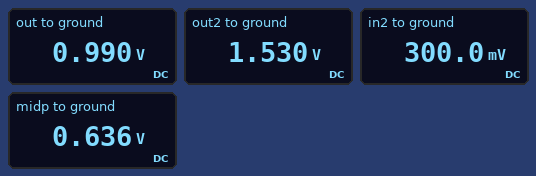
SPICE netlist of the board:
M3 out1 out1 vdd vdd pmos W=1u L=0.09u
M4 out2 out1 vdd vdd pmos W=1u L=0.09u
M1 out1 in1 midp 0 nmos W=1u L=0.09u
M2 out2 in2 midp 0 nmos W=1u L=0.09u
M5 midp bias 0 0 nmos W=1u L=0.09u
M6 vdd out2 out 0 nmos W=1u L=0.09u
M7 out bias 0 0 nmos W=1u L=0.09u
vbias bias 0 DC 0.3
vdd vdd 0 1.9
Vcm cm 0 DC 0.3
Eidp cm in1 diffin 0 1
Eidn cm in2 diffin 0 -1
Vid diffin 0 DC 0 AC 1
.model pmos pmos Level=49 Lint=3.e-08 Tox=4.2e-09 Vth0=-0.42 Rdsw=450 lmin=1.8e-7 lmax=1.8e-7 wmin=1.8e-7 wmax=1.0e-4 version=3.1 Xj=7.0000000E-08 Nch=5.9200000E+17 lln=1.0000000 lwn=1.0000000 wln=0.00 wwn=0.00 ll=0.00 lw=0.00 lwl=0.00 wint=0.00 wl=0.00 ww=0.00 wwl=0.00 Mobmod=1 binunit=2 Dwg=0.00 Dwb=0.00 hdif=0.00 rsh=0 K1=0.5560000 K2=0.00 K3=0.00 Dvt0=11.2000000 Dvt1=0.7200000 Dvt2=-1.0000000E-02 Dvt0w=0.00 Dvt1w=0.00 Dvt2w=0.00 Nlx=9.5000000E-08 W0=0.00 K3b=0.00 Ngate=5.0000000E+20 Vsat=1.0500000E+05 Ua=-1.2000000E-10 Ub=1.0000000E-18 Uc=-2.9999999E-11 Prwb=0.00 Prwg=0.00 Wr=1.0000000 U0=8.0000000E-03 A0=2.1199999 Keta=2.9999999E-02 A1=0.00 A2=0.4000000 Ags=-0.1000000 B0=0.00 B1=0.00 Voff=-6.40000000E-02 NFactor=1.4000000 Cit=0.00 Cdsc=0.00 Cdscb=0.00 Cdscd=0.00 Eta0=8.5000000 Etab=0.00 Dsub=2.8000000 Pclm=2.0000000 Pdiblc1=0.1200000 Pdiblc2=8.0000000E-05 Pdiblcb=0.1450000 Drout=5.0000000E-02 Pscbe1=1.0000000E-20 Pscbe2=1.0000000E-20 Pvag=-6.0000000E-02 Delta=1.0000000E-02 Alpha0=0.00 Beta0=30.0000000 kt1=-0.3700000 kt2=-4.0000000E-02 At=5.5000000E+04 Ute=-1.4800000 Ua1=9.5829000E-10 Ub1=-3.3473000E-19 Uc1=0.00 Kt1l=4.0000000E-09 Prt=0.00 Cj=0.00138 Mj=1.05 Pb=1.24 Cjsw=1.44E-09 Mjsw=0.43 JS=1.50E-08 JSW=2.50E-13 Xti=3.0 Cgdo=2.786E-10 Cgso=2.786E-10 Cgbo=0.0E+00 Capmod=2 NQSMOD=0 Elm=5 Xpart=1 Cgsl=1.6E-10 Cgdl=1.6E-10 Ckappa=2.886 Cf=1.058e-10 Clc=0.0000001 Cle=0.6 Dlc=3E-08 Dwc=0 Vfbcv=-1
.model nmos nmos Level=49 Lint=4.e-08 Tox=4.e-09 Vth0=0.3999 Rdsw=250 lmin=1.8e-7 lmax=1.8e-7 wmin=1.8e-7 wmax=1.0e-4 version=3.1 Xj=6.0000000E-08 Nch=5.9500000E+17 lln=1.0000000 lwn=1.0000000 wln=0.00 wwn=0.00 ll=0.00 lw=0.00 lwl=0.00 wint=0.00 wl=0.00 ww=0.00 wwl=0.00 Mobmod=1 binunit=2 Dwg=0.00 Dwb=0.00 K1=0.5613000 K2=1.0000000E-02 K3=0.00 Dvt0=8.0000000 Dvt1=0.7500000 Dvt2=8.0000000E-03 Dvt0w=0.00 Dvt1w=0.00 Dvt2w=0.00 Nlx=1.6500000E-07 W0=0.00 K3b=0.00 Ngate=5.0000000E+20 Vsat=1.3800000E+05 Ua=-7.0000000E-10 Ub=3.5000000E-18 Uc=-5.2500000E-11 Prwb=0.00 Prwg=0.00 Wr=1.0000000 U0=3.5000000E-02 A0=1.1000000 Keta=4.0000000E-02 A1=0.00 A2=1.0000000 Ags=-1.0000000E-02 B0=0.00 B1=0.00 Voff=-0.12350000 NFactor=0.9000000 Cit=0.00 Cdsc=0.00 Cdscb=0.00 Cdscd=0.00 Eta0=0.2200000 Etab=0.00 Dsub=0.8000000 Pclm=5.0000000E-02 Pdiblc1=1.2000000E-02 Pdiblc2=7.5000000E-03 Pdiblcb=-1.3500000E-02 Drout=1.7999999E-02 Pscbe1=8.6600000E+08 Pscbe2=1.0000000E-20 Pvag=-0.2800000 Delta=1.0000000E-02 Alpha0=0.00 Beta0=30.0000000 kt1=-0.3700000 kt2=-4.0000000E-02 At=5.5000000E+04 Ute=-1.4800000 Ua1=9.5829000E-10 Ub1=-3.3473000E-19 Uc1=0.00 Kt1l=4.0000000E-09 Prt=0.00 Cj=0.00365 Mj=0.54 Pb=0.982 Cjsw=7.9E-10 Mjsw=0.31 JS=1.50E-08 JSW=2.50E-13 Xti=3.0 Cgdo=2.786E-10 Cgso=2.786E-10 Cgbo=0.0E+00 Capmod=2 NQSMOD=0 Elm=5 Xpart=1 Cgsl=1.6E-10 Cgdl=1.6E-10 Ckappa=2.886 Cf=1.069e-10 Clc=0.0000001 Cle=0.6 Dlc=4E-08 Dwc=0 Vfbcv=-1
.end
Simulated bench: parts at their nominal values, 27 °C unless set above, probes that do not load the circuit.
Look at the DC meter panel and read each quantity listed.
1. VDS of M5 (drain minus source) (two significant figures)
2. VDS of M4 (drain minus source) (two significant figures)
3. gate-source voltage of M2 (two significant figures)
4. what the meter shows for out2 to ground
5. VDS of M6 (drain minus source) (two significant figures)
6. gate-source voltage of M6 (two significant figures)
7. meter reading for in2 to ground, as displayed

640 mV
-370 mV
-340 mV
1.530 V
910 mV
540 mV
300.0 mV
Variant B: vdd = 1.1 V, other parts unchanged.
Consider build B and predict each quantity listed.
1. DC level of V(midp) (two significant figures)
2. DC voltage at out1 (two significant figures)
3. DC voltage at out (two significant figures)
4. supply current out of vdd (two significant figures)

420 mV
800 mV
520 mV
1.5 mA
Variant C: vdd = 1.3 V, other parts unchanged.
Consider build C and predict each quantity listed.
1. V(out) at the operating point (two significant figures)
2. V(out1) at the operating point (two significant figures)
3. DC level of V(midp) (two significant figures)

630 mV
980 mV
480 mV
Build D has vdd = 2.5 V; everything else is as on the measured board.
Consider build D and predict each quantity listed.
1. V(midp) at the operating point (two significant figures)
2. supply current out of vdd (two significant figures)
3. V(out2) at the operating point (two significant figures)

780 mV
2.5 mA
2.1 V
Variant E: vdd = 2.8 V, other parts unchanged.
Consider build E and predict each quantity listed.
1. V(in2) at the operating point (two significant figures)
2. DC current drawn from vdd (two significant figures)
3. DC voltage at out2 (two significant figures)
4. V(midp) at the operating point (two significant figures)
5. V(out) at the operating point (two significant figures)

300 mV
2.7 mA
2.4 V
850 mV
1.5 V
